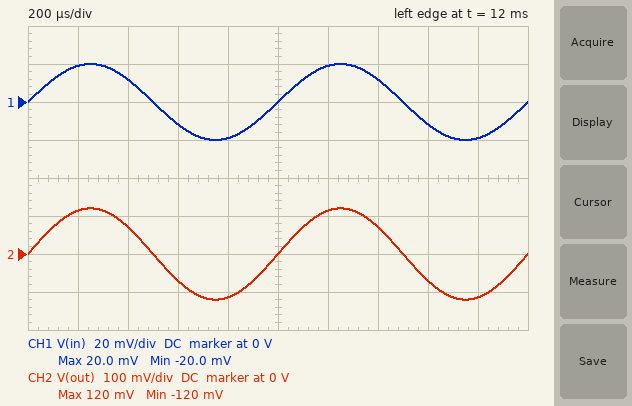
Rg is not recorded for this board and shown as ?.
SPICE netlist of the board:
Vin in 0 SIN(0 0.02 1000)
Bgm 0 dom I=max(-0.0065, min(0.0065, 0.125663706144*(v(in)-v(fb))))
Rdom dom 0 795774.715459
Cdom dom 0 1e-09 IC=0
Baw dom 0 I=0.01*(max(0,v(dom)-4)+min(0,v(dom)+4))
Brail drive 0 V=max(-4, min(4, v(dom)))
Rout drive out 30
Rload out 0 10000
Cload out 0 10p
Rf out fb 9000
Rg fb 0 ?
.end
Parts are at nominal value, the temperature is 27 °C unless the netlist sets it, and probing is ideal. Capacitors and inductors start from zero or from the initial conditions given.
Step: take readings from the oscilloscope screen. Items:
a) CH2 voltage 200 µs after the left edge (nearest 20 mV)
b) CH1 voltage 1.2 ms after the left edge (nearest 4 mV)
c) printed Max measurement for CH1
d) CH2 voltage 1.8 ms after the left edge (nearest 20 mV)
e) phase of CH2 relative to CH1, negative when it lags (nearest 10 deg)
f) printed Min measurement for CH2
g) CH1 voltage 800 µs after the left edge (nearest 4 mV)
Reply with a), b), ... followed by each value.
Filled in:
a) 120 mV
b) 20 mV
c) 20.0 mV
d) -120 mV
e) 0 deg
f) -120 mV
g) -20 mV
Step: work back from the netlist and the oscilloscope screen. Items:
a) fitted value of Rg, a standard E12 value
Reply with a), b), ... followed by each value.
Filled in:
a) 1.8 kΩ
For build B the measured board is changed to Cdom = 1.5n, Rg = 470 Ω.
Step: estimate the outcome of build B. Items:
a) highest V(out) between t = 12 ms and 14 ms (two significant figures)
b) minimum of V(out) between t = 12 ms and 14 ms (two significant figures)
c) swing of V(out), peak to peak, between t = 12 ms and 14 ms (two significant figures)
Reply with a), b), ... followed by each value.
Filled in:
a) 400 mV
b) -400 mV
c) 810 mV
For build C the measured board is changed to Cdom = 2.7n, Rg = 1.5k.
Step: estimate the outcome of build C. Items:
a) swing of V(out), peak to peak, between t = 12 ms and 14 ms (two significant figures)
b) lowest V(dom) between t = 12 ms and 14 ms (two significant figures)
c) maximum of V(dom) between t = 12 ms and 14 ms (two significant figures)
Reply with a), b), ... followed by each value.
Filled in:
a) 280 mV
b) -140 mV
c) 140 mV
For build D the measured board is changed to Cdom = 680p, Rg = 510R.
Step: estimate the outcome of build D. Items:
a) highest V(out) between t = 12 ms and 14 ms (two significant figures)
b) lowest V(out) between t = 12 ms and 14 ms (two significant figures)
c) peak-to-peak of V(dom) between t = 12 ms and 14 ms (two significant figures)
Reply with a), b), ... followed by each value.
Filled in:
a) 370 mV
b) -370 mV
c) 750 mV
